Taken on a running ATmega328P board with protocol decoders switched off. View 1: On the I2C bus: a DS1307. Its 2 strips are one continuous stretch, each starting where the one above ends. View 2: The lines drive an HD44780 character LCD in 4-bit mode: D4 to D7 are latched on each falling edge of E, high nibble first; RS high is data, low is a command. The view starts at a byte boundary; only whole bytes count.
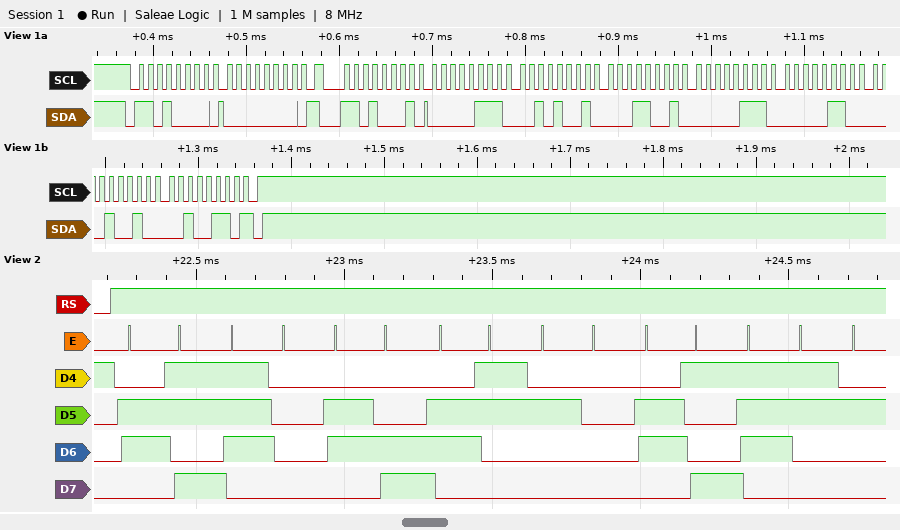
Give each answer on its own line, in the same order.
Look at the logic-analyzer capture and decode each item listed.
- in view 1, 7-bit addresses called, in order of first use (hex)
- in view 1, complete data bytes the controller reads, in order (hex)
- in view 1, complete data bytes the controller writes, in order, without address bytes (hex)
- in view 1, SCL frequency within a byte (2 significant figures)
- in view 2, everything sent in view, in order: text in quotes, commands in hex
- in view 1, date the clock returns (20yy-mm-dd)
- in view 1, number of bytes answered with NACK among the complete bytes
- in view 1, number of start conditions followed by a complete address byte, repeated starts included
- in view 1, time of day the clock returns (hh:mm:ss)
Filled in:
0x68
07 29 19 07 06 12 26
00
100 kHz
"kplc is"
2026-12-06
1
2
19:29:07
